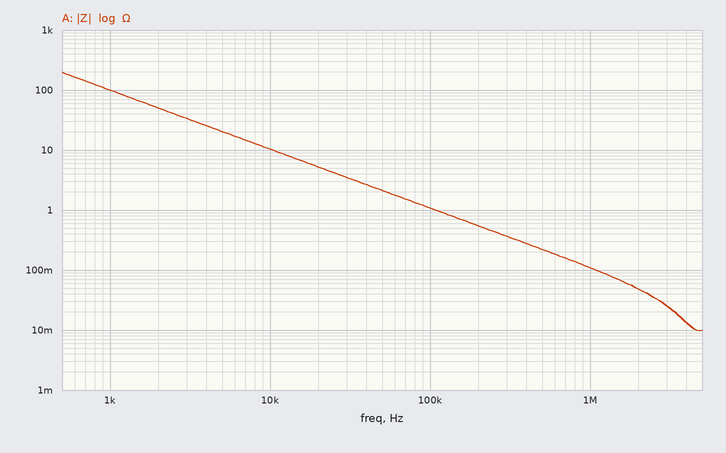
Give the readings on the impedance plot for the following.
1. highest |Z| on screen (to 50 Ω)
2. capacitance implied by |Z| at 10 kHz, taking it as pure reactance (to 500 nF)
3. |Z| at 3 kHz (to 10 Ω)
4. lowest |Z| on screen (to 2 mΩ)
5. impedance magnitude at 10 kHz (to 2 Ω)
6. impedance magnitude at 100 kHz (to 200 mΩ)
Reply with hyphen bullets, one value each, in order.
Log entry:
- 200 Ω
- 1.5 µF
- 30 Ω
- 10 mΩ
- 10 Ω
- 1.0 Ω
